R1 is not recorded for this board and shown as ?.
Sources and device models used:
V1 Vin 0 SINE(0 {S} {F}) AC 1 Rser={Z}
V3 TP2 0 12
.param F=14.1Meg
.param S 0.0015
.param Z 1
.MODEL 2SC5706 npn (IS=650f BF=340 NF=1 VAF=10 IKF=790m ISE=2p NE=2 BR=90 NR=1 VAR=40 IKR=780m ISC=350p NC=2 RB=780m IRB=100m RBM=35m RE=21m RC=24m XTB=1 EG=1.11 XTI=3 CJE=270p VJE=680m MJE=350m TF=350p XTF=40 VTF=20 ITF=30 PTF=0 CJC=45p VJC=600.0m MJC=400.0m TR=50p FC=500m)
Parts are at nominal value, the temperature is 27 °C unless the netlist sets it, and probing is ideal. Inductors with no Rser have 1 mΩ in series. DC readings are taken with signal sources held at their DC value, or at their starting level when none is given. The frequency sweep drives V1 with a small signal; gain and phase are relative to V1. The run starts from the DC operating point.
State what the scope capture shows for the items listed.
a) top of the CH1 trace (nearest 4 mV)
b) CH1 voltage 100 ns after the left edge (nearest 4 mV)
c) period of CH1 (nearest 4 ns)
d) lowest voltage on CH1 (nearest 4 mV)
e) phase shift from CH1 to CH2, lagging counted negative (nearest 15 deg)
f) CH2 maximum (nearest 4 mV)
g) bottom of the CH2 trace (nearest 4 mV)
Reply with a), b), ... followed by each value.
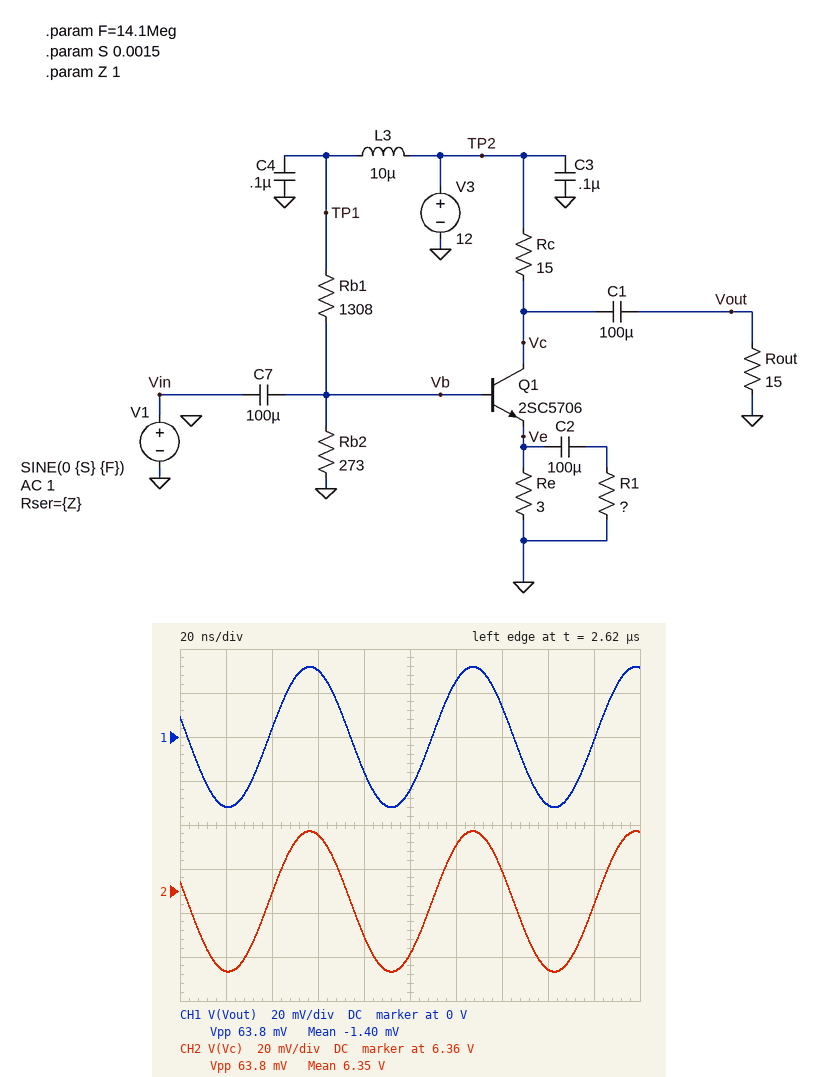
a) 32 mV
b) -24 mV
c) 72 ns
d) -32 mV
e) 0 deg
f) 6.388 V
g) 6.324 V
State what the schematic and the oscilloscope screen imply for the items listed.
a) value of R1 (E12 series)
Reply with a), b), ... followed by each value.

a) 0.22 Ω
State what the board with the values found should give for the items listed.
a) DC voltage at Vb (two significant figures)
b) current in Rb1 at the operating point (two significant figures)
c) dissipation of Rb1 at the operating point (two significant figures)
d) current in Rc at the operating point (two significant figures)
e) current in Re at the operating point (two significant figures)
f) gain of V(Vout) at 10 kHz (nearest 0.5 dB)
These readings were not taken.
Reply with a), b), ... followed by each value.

a) 1.8 V
b) 7.8 mA
c) 79 mW
d) 380 mA
e) 380 mA
f) 26.0 dB
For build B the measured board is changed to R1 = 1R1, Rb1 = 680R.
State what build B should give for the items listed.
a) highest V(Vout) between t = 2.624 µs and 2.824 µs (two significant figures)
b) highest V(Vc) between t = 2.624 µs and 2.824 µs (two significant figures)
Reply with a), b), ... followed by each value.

a) 11 mV
b) 2.3 V
